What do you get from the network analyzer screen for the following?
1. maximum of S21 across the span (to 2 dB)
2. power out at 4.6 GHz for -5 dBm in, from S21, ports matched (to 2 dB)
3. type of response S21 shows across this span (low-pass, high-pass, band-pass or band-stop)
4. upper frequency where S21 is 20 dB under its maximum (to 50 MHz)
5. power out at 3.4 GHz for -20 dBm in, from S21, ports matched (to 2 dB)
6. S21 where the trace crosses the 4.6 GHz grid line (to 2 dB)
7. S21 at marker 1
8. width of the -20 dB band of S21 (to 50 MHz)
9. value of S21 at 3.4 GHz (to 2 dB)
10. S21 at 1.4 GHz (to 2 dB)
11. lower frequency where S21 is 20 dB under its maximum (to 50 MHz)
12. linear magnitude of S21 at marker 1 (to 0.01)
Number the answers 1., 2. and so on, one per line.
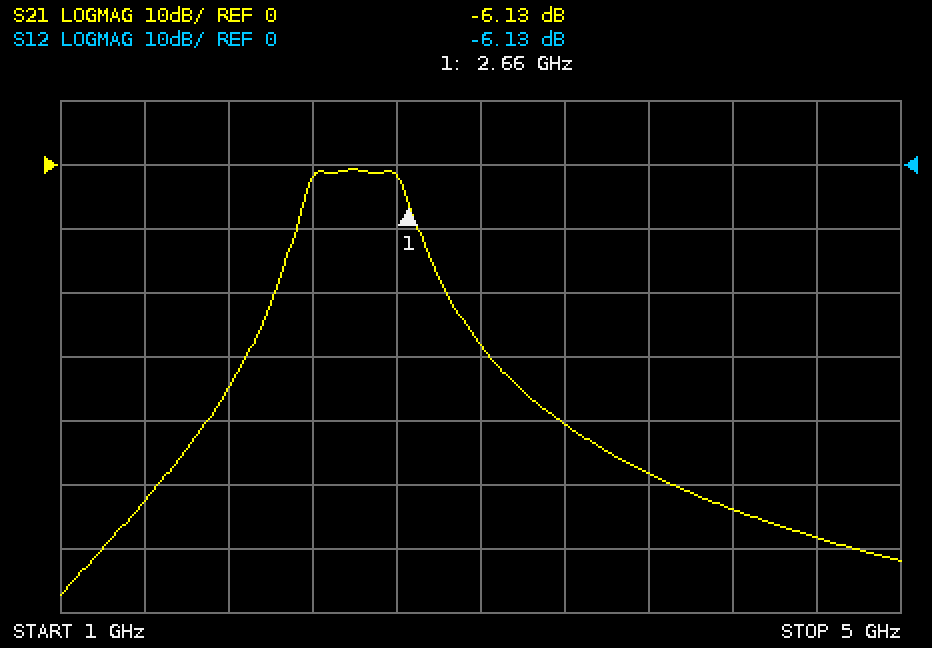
1. 0 dB
2. -64 dBm
3. band-pass
4. 2.85 GHz
5. -60 dBm
6. -58 dB
7. -6.13 dB
8. 850 MHz
9. -40 dB
10. -52 dB
11. 2.00 GHz
12. 0.49
